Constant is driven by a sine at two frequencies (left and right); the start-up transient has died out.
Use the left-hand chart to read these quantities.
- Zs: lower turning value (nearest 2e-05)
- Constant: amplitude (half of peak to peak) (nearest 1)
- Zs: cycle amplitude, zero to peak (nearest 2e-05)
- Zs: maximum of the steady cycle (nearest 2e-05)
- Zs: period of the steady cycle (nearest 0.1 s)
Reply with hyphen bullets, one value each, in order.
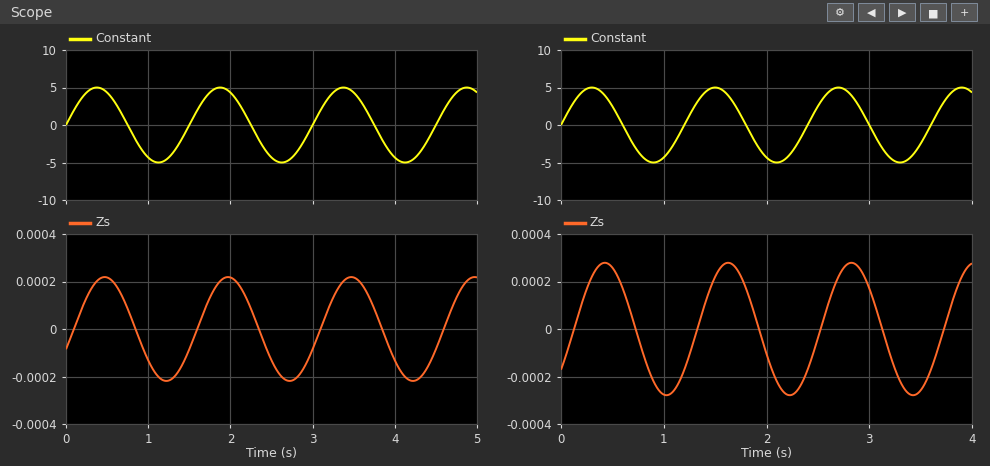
- -0.00022
- 5
- 0.00022
- 0.00022
- 1.5 s
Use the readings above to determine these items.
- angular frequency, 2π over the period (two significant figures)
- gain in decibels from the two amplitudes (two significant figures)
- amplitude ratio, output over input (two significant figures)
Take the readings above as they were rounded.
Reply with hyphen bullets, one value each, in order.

- 4.2 rad/s
- -87 dB
- 0.000044
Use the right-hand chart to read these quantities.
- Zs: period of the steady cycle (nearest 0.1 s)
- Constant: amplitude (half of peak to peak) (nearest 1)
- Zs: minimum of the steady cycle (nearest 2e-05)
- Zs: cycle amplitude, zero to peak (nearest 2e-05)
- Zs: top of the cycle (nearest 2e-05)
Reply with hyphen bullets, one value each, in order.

- 1.2 s
- 5
- -0.00028
- 0.00028
- 0.00028
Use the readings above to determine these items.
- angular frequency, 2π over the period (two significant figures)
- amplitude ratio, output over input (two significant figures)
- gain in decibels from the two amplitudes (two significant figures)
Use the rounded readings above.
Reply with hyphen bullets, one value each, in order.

- 5.2 rad/s
- 0.000056
- -85 dB
